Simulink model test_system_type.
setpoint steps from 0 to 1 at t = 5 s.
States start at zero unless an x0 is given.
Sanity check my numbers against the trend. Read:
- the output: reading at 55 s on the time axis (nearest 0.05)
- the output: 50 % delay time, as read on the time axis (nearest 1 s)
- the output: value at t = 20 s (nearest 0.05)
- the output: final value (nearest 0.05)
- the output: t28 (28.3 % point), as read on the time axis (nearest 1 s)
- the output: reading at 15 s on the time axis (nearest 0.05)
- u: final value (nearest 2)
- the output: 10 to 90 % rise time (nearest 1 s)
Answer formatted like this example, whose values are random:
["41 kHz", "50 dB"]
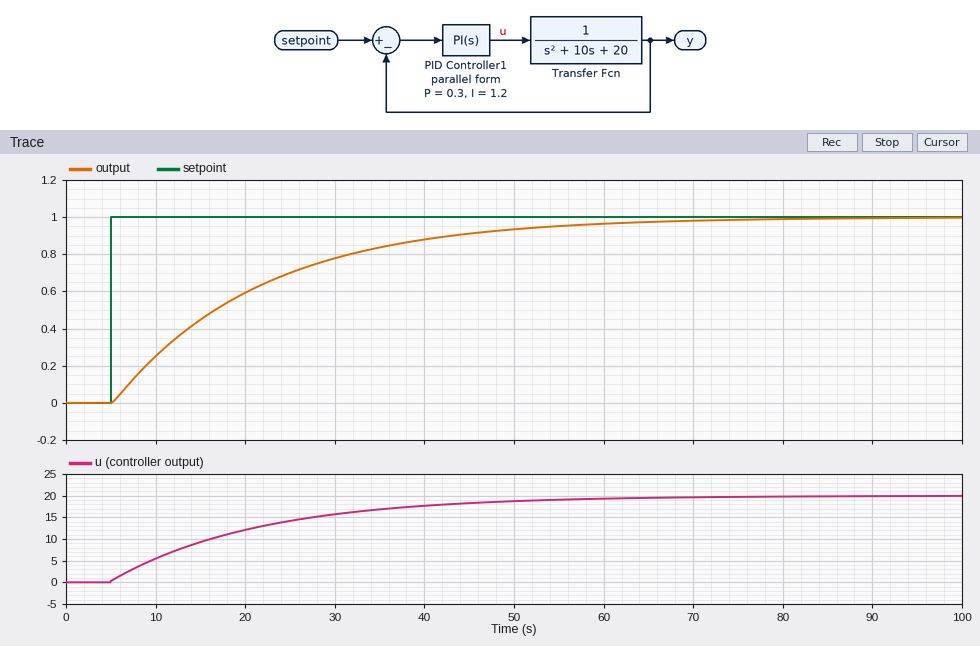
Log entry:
["0.95", "17 s", "0.60", "1.00", "11 s", "0.45", "20", "36 s"]
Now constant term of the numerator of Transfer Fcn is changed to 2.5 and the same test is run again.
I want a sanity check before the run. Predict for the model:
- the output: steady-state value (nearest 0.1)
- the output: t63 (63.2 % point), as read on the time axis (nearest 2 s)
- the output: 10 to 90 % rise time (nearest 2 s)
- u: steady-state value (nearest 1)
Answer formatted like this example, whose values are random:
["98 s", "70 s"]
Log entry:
["1.0", "12 s", "14 s", "8"]
